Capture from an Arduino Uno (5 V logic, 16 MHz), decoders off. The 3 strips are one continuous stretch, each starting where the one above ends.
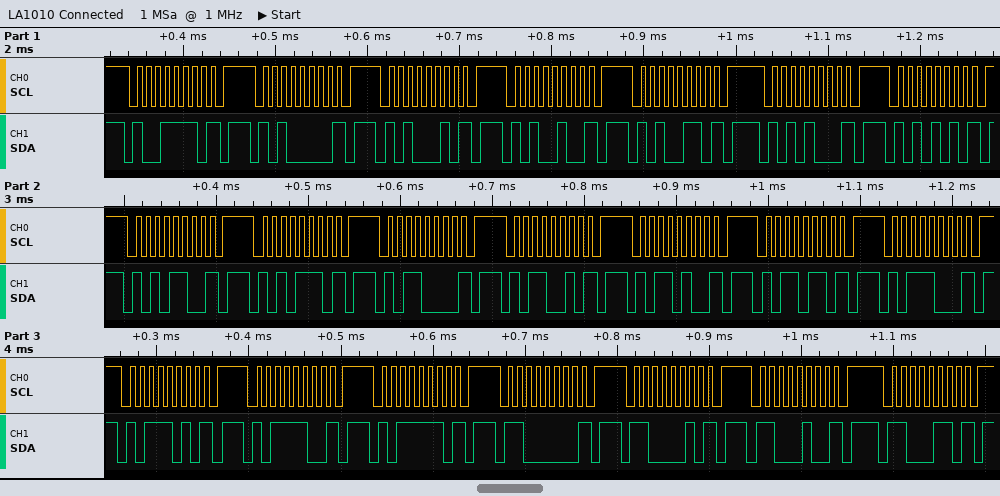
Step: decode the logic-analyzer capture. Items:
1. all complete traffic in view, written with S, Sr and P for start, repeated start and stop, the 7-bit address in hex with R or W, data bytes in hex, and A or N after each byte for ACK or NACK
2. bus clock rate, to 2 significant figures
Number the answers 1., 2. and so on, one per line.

1. S 4FW N P S 50W N P S 51W N P S 52W N P S 53W N P S 54W N P S 55W N P S 56W N P S 57W N P S 58W N P S 59W N P S 5AW N P S 5BW N P S 5CW N P S 5DW N P S 5EW N P S 5FW N P S 60W N P S 61W N P S 62W N P S 63W N P
2. 100 kHz
